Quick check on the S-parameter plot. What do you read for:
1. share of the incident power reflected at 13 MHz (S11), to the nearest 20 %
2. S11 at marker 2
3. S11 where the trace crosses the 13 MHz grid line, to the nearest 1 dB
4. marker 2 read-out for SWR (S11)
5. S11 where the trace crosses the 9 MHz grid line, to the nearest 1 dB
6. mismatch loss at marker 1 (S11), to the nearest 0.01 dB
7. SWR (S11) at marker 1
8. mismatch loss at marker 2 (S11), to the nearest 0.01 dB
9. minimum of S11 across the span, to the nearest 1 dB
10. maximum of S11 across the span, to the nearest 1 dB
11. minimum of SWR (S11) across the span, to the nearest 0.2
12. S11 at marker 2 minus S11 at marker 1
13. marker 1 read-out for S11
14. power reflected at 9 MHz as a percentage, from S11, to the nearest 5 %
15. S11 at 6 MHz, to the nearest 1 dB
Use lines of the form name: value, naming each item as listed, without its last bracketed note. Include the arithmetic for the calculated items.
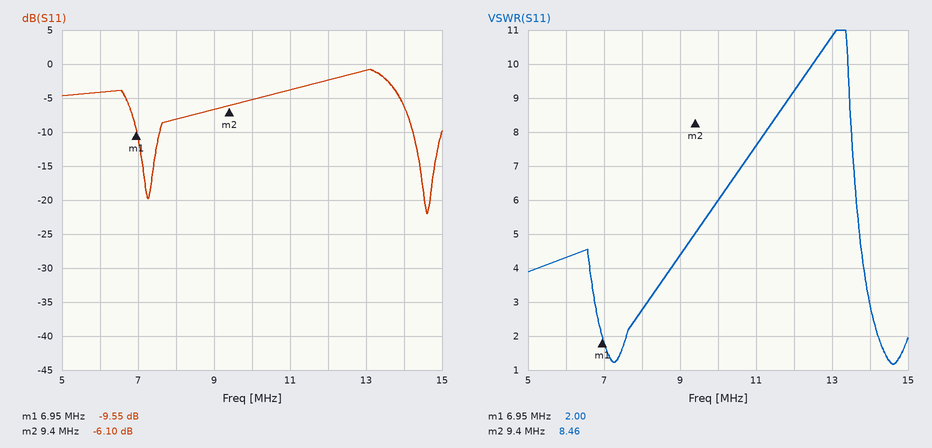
share of the incident power reflected at 13 MHz (S11), to the nearest 20 %: 10^(-1/10) ≈ 79.4 %, so 80 % to the nearest 20 %
S11 at marker 2: -6.10 dB
S11 where the trace crosses the 13 MHz grid line, to the nearest 1 dB: -1 dB
marker 2 read-out for SWR: 8.46
S11 where the trace crosses the 9 MHz grid line, to the nearest 1 dB: -7 dB
mismatch loss at marker 1 (S11), to the nearest 0.01 dB: −10 log10(1 − 10^(-9.55/10)) ≈ 0.51 dB
SWR (S11) at marker 1: 2.00
mismatch loss at marker 2 (S11), to the nearest 0.01 dB: −10 log10(1 − 10^(-6.1/10)) ≈ 1.22 dB
minimum of S11 across the span, to the nearest 1 dB: -22 dB
maximum of S11 across the span, to the nearest 1 dB: -1 dB
minimum of SWR (S11) across the span, to the nearest 0.2: 1.2
S11 at marker 2 minus S11 at marker 1: -6.1 − (-9.55) = 3.45 dB
marker 1 read-out for S11: -9.55 dB
power reflected at 9 MHz as a percentage, from S11, to the nearest 5 %: 10^(-7/10) ≈ 20 %
S11 at 6 MHz, to the nearest 1 dB: -4 dB
